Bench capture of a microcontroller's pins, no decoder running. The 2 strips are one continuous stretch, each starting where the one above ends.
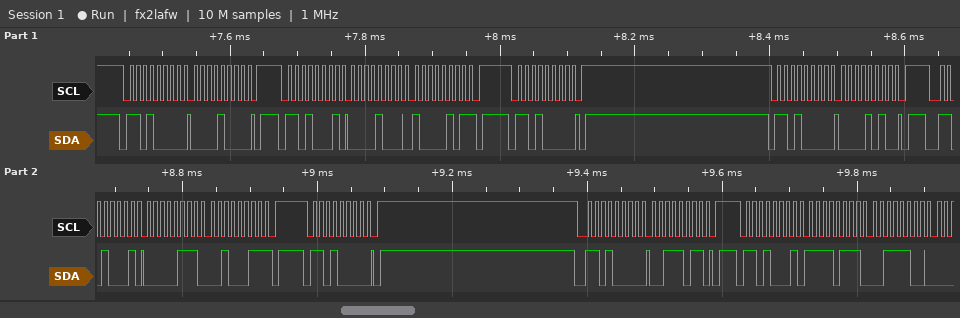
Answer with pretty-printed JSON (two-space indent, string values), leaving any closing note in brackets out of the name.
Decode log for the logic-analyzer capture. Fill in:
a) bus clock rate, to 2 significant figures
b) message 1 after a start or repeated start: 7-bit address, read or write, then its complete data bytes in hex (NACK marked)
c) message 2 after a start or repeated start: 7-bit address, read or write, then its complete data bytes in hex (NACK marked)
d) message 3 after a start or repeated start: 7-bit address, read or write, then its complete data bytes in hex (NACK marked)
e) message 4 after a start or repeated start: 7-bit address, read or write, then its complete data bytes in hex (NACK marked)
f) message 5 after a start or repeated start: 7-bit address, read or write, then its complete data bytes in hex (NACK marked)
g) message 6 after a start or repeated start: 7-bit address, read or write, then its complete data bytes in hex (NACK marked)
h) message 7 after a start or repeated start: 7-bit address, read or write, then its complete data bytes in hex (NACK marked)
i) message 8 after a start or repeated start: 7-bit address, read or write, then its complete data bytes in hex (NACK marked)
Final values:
{
  "bus clock rate, to 2 significant figures": "100 kHz",
  "message 1 after a start or repeated start: 7-bit address, read or write, then its complete data bytes in hex": "0x68 write: 08",
  "message 2 after a start or repeated start: 7-bit address, read or write, then its complete data bytes in hex": "0x68 read: 08 85 NACK",
  "message 3 after a start or repeated start: 7-bit address, read or write, then its complete data bytes in hex": "0x68 write",
  "message 4 after a start or repeated start: 7-bit address, read or write, then its complete data bytes in hex": "0x68 write: 0A",
  "message 5 after a start or repeated start: 7-bit address, read or write, then its complete data bytes in hex": "0x68 read: 07 23 NACK",
  "message 6 after a start or repeated start: 7-bit address, read or write, then its complete data bytes in hex": "0x68 write",
  "message 7 after a start or repeated start: 7-bit address, read or write, then its complete data bytes in hex": "0x68 write: 3B",
  "message 8 after a start or repeated start: 7-bit address, read or write, then its complete data bytes in hex": "0x68 read: F7 3C"
}
